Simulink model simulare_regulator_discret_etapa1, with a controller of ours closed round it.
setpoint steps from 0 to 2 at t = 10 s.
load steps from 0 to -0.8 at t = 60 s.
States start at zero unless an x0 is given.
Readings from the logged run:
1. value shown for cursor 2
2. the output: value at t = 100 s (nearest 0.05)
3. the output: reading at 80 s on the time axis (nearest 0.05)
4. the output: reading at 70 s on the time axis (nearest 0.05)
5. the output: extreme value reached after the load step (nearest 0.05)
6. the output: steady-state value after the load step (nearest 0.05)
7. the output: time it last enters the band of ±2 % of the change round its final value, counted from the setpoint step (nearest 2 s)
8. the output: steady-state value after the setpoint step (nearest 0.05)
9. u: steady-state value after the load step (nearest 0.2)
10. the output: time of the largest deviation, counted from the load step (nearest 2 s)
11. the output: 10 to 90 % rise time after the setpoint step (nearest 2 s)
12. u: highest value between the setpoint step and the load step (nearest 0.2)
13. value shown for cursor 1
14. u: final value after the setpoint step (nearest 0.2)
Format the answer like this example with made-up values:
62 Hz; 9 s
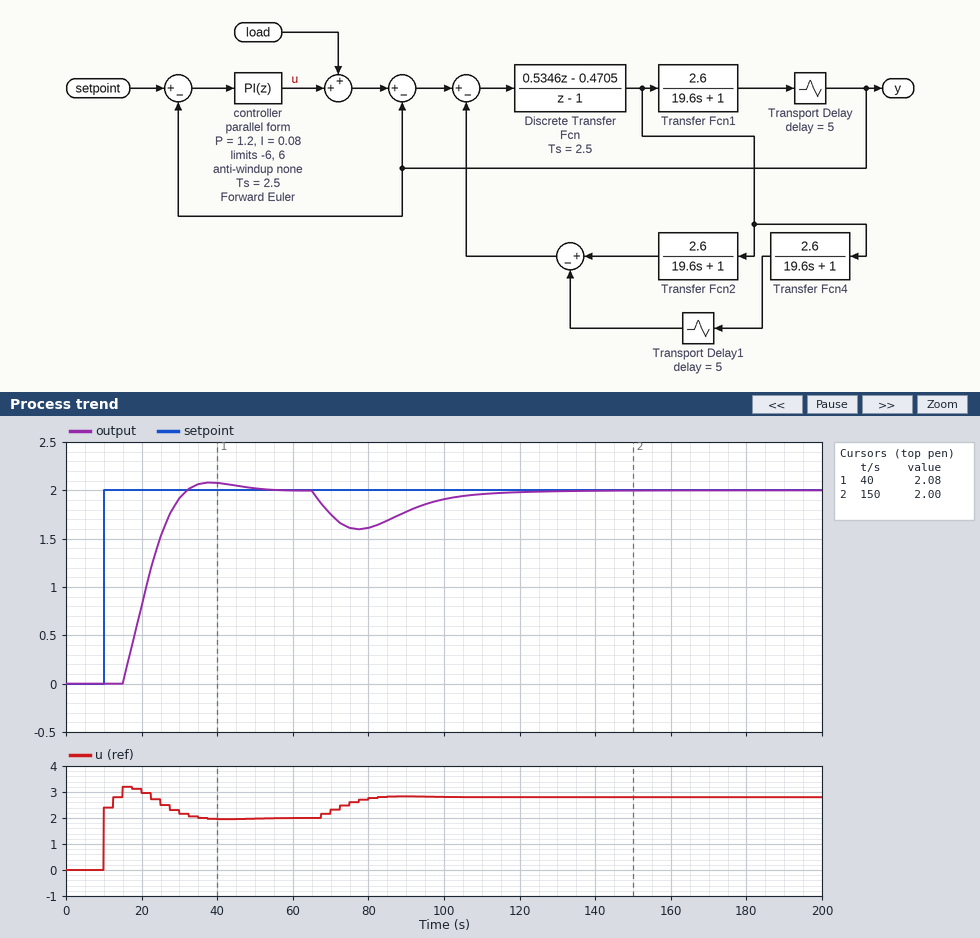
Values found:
2.00; 1.90; 1.60; 1.75; 1.60; 2.00; 36 s; 2.00; 2.8; 18 s; 12 s; 3.2; 2.08; 2.0
